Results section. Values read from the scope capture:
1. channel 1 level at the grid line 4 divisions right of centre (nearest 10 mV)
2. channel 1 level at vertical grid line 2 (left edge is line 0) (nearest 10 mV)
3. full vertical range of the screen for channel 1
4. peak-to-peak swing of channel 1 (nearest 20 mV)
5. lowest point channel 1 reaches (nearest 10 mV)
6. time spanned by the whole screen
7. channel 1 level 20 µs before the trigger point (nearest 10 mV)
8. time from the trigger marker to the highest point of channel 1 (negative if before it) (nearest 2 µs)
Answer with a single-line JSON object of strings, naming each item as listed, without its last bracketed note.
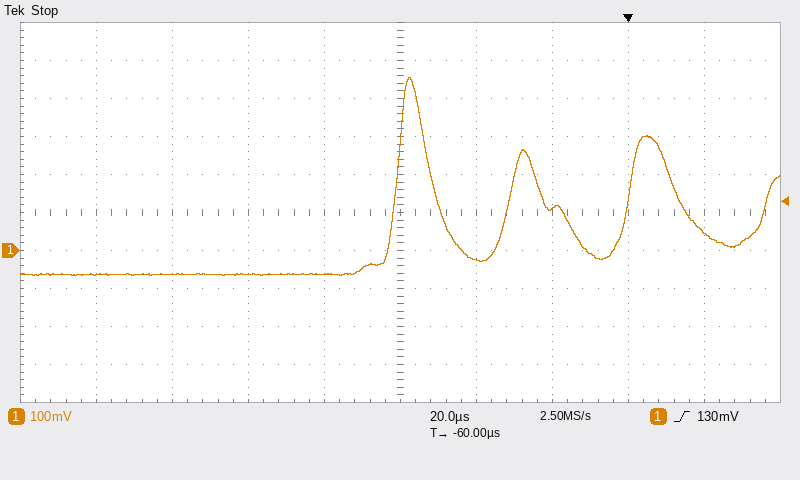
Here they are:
{"channel 1 level at the grid line 4 divisions right of centre": "50 mV", "channel 1 level at vertical grid line 2 (left edge is line 0)": "-60 mV", "full vertical range of the screen for channel 1": "1 V", "peak-to-peak swing of channel 1": "520 mV", "lowest point channel 1 reaches": "-70 mV", "time spanned by the whole screen": "200 µs", "channel 1 level 20 µs before the trigger point": "110 mV", "time from the trigger marker to the highest point of channel 1 (negative if before it)": "-58 µs"}
